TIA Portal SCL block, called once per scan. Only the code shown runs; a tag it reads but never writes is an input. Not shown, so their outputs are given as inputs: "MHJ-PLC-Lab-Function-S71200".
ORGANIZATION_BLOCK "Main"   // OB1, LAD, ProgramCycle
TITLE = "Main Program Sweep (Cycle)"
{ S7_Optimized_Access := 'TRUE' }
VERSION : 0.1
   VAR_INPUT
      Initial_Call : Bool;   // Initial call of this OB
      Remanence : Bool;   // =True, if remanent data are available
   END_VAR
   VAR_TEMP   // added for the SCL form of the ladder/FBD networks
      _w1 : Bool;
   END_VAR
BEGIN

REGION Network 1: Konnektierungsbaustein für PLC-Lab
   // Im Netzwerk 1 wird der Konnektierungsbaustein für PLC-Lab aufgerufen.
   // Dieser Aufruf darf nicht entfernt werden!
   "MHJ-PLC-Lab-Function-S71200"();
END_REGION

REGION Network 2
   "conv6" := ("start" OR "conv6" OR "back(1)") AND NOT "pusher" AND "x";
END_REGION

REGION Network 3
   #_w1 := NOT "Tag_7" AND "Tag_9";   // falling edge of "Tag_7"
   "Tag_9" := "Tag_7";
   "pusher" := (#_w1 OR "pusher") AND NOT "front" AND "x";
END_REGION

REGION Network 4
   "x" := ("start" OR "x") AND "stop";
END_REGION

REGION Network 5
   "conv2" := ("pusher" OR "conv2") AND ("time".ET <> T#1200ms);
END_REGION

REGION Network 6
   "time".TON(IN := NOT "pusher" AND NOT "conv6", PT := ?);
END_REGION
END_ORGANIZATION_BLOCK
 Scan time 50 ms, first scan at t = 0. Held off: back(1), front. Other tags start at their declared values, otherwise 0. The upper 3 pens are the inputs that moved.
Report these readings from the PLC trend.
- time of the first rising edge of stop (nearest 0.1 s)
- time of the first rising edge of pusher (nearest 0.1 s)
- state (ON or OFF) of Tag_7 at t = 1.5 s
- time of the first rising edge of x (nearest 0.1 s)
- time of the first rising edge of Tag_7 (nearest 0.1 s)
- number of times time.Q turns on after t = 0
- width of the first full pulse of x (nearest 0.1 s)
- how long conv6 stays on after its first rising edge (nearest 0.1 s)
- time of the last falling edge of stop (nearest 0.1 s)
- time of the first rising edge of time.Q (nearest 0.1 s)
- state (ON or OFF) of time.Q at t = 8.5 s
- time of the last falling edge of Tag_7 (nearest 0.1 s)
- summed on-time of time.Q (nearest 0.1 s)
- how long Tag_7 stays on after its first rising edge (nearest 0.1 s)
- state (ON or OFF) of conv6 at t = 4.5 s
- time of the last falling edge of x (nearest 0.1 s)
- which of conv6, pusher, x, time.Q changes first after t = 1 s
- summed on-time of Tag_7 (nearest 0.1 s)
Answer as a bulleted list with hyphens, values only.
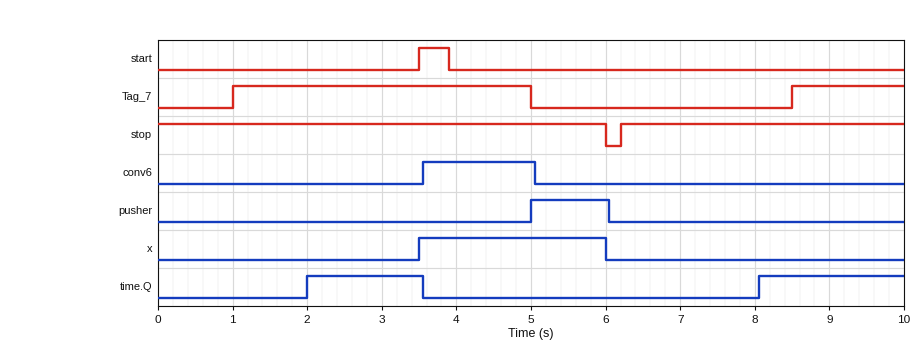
- 6.2 s
- 5.0 s
- ON
- 3.5 s
- 1.0 s
- 2
- 2.5 s
- 1.5 s
- 6.0 s
- 2.0 s
- ON
- 5.0 s
- 3.5 s
- 4.0 s
- ON
- 6.0 s
- time.Q
- 5.5 s
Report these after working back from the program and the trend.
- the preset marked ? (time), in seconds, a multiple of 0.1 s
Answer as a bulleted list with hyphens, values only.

- 2.0 s
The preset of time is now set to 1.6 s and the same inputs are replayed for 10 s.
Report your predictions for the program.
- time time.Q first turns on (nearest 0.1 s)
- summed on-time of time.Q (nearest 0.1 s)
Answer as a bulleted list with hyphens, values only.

- 1.6 s
- 4.3 s
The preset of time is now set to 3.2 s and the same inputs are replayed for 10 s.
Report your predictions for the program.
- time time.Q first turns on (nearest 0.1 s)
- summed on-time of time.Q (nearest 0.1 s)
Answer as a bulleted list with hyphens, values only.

- 3.2 s
- 1.1 s
